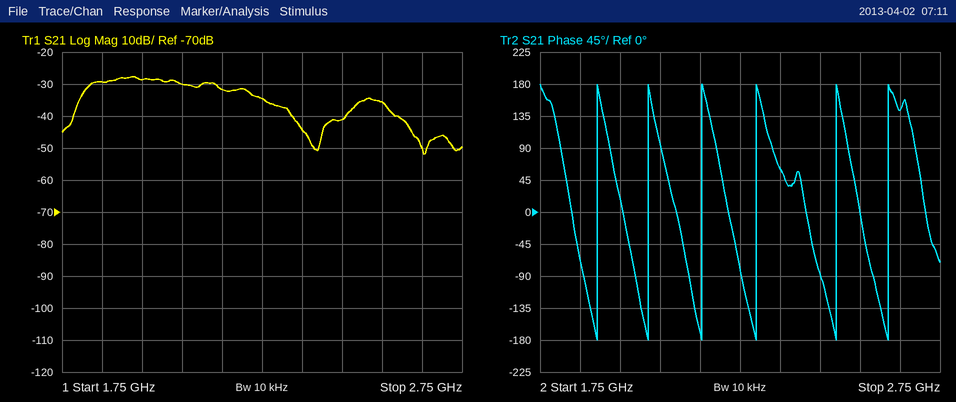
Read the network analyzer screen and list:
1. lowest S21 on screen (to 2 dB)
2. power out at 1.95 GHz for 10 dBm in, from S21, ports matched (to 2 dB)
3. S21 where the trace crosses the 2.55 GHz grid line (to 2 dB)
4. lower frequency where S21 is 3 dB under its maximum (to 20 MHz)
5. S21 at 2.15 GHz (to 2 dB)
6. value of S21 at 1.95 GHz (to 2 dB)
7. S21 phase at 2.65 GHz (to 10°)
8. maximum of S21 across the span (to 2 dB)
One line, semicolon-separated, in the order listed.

-52 dB; -18 dBm; -36 dB; 1.82 GHz; -32 dB; -28 dB; 140°; -28 dB
